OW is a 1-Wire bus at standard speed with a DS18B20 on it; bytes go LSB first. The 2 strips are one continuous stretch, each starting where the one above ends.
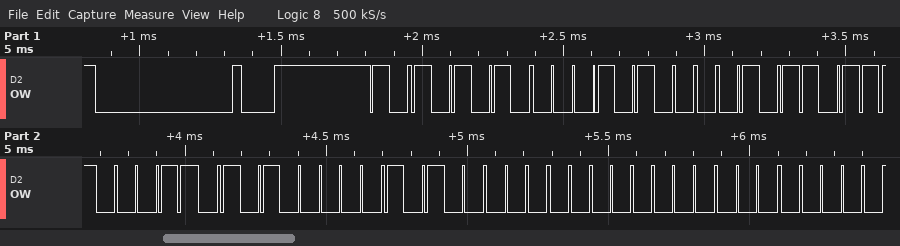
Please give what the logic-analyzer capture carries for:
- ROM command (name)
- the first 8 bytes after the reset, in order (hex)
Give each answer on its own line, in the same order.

Match ROM
55 28 B4 63 05 05 00 00
